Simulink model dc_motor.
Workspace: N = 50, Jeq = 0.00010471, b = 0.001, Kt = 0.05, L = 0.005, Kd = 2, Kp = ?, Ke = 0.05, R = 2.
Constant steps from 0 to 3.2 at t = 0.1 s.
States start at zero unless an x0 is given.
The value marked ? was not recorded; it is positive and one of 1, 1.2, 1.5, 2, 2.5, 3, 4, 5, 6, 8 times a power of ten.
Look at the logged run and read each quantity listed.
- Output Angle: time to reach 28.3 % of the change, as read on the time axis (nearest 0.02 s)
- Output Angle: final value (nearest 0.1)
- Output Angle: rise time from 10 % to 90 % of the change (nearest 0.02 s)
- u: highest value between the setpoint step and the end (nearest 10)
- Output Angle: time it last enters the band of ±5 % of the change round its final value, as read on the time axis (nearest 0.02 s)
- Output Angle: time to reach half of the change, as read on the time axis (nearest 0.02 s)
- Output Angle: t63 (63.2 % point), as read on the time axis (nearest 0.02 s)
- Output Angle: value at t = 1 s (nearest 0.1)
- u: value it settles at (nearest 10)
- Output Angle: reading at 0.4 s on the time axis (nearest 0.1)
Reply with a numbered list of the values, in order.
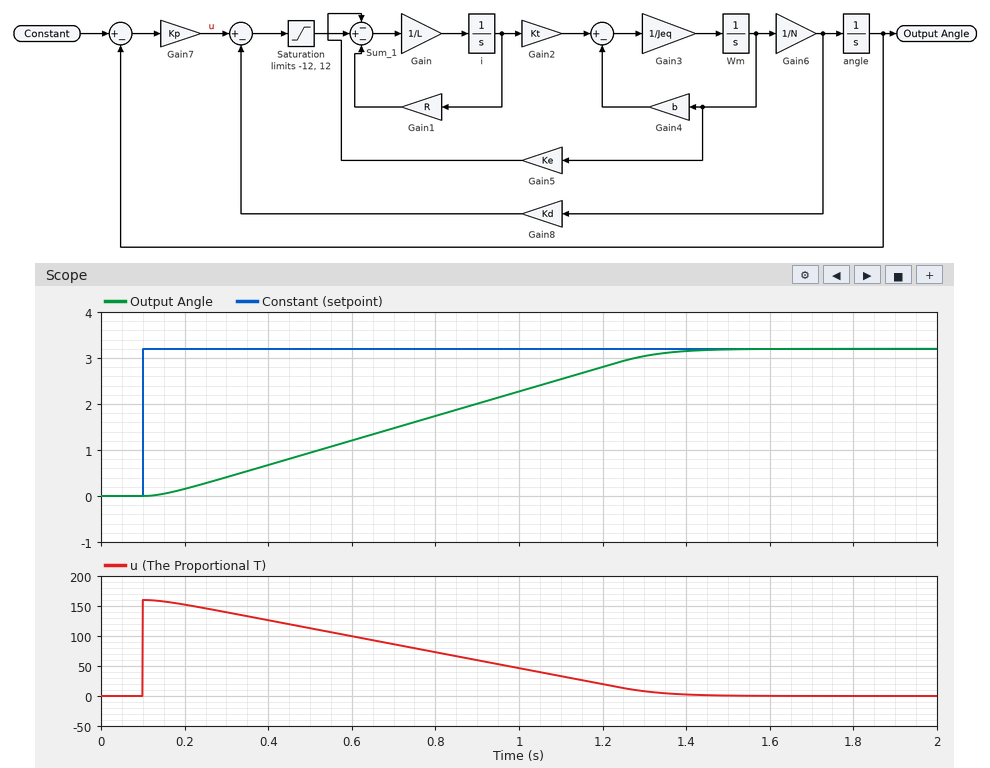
1. 0.48 s
2. 3.2
3. 0.96 s
4. 160
5. 1.30 s
6. 0.74 s
7. 0.90 s
8. 2.3
9. 0
10. 0.7
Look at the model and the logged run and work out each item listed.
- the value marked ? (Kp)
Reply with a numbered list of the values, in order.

1. 50
